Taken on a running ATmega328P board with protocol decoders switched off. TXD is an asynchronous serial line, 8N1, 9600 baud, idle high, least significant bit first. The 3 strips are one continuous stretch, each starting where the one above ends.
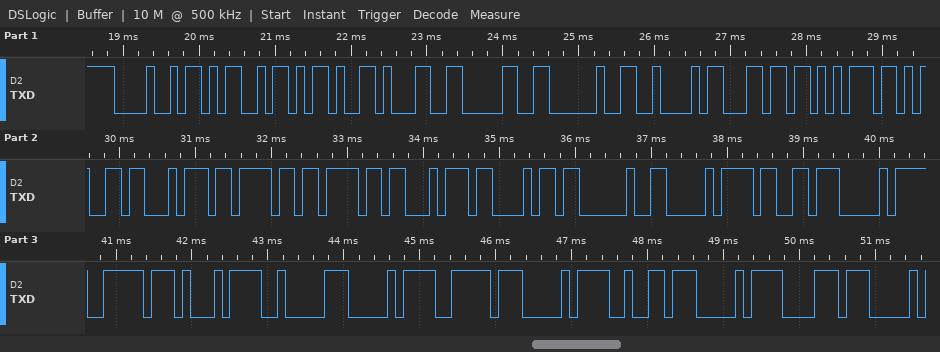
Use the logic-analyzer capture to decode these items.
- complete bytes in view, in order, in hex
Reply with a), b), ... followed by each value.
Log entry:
a) 48 4D 2D 31 30 20 42 6C 75 65 74 6F 6F 74 68 20 D0 B3 D0 BE D1 82 D0 BE D0 B2 D0 B8
